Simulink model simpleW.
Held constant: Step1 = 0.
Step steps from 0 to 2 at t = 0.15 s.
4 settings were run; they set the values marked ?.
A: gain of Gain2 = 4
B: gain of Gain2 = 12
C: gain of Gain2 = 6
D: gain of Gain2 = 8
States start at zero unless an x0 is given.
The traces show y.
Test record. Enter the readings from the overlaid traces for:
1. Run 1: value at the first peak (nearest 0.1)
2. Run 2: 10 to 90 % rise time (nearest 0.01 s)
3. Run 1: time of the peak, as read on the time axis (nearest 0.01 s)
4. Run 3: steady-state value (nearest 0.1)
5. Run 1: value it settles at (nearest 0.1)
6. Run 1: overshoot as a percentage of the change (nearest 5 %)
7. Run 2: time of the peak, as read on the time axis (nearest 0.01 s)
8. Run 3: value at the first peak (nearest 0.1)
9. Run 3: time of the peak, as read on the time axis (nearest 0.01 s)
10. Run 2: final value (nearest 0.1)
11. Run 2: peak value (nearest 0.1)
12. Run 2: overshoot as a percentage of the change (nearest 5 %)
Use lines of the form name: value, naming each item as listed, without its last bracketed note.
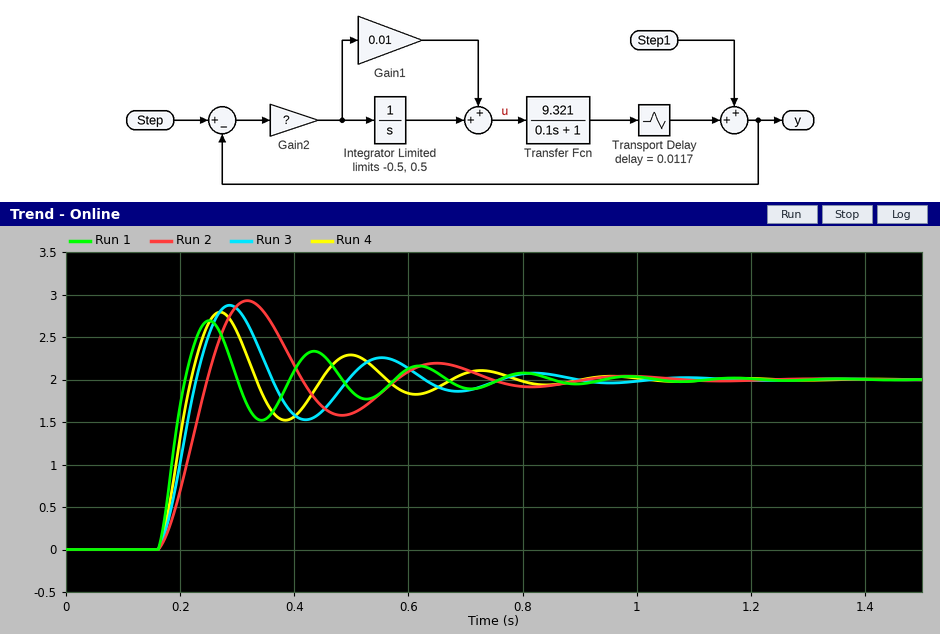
Run 1: value at the first peak: 2.7
Run 2: 10 to 90 % rise time: 0.06 s
Run 1: time of the peak, as read on the time axis: 0.25 s
Run 3: steady-state value: 2.0
Run 1: value it settles at: 2.0
Run 1: overshoot as a percentage of the change: 35 %
Run 2: time of the peak, as read on the time axis: 0.32 s
Run 3: value at the first peak: 2.9
Run 3: time of the peak, as read on the time axis: 0.29 s
Run 2: final value: 2.0
Run 2: peak value: 2.9
Run 2: overshoot as a percentage of the change: 45 %
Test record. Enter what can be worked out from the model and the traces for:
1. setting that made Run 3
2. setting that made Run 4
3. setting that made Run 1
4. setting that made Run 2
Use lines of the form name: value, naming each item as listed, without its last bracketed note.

setting that made Run 3: C
setting that made Run 4: D
setting that made Run 1: B
setting that made Run 2: A
